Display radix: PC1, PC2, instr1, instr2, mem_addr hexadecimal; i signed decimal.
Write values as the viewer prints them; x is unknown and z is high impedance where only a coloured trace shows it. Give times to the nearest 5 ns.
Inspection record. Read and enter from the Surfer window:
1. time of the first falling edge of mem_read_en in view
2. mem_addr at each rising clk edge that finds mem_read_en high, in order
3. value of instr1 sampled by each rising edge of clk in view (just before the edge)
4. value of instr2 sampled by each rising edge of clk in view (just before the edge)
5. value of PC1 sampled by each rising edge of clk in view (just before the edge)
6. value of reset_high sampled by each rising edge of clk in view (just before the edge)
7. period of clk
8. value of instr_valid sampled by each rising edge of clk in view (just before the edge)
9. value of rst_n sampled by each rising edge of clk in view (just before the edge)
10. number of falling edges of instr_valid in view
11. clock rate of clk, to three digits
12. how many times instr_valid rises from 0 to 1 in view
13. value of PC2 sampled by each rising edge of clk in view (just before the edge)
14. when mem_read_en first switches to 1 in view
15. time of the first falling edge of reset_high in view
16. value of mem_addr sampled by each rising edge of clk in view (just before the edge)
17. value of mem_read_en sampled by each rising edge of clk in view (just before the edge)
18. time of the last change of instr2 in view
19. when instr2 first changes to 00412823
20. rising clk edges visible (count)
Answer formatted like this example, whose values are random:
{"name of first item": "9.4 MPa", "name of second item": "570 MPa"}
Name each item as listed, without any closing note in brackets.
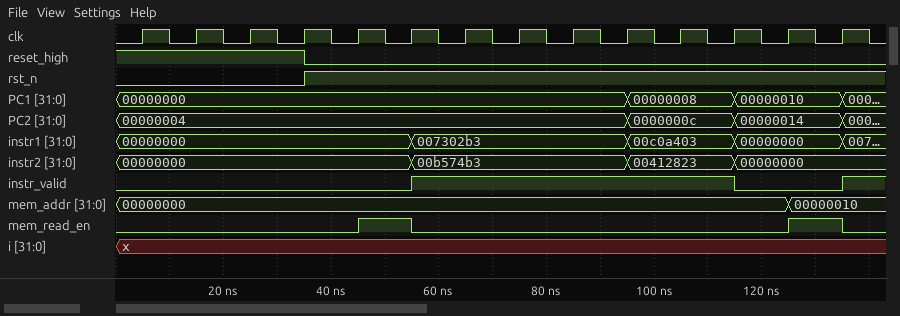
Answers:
{"time of the first falling edge of mem_read_en in view": "55 ns", "mem_addr at each rising clk edge that finds mem_read_en high, in order": "00000000, 00000010", "value of instr1 sampled by each rising edge of clk in view": "00000000, 00000000, 00000000, 00000000, 00000000, 00000000, 007302b3, 007302b3, 007302b3, 007302b3, 00c0a403, 00c0a403, 00000000, 00000000", "value of instr2 sampled by each rising edge of clk in view": "00000000, 00000000, 00000000, 00000000, 00000000, 00000000, 00b574b3, 00b574b3, 00b574b3, 00b574b3, 00412823, 00412823, 00000000, 00000000", "value of PC1 sampled by each rising edge of clk in view": "00000000, 00000000, 00000000, 00000000, 00000000, 00000000, 00000000, 00000000, 00000000, 00000000, 00000008, 00000008, 00000010, 00000010", "value of reset_high sampled by each rising edge of clk in view": "1 1 1 1 0 0 0 0 0 0 0 0 0 0", "period of clk": "10 ns", "value of instr_valid sampled by each rising edge of clk in view": "0 0 0 0 0 0 1 1 1 1 1 1 0 0", "value of rst_n sampled by each rising edge of clk in view": "0 0 0 0 1 1 1 1 1 1 1 1 1 1", "number of falling edges of instr_valid in view": "1", "clock rate of clk, to three digits": "100 MHz", "how many times instr_valid rises from 0 to 1 in view": "2", "value of PC2 sampled by each rising edge of clk in view": "00000004, 00000004, 00000004, 00000004, 00000004, 00000004, 00000004, 00000004, 00000004, 00000004, 0000000c, 0000000c, 00000014, 00000014", "when mem_read_en first switches to 1 in view": "45 ns", "time of the first falling edge of reset_high in view": "35 ns", "value of mem_addr sampled by each rising edge of clk in view": "00000000, 00000000, 00000000, 00000000, 00000000, 00000000, 00000000, 00000000, 00000000, 00000000, 00000000, 00000000, 00000000, 00000010", "value of mem_read_en sampled by each rising edge of clk in view": "0 0 0 0 0 1 0 0 0 0 0 0 0 1", "time of the last change of instr2 in view": "115 ns", "when instr2 first changes to 00412823": "95 ns", "rising clk edges visible": "14"}
